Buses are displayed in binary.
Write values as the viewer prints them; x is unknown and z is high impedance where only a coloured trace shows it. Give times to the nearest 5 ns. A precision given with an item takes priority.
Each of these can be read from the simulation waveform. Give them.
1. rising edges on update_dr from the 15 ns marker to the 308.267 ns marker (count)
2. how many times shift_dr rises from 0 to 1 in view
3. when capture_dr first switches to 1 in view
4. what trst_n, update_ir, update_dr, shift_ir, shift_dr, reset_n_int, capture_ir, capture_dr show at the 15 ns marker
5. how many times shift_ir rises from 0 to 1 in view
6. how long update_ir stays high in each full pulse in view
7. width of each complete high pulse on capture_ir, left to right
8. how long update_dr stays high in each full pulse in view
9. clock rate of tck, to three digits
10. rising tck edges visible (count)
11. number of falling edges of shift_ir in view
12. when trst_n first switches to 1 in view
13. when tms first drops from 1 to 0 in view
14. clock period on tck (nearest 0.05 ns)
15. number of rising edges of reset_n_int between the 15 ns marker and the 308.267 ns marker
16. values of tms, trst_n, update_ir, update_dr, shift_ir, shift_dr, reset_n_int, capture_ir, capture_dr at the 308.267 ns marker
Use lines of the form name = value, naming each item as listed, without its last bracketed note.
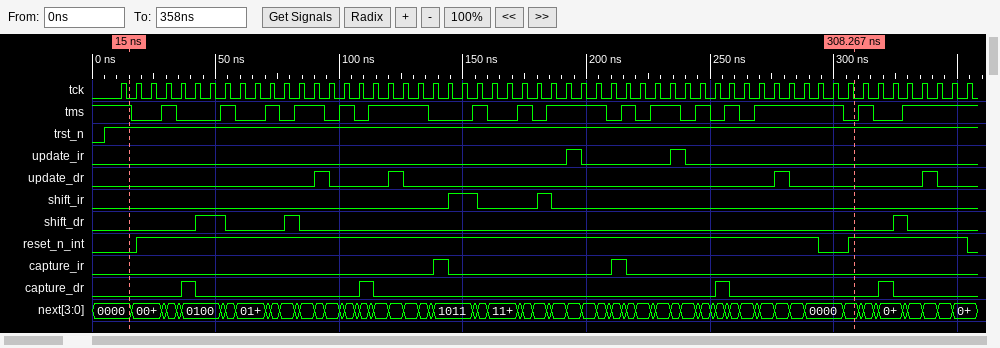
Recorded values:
rising edges on update_dr from the 15 ns marker to the 308.267 ns marker = 3
how many times shift_dr rises from 0 to 1 in view = 3
when capture_dr first switches to 1 in view = 35 ns
what trst_n, update_ir, update_dr, shift_ir, shift_dr, reset_n_int, capture_ir, capture_dr show at the 15 ns marker = trst_n=1, update_ir=0, update_dr=0, shift_ir=0, shift_dr=0, reset_n_int=0, capture_ir=0, capture_dr=0
how many times shift_ir rises from 0 to 1 in view = 2
how long update_ir stays high in each full pulse in view = 5 ns, 5 ns
width of each complete high pulse on capture_ir, left to right = 5 ns, 5 ns
how long update_dr stays high in each full pulse in view = 5 ns, 5 ns, 5 ns, 5 ns
clock rate of tck, to three digits = 167 MHz
rising tck edges visible = 58
number of falling edges of shift_ir in view = 2
when trst_n first switches to 1 in view = 5 ns
when tms first drops from 1 to 0 in view = 15 ns
clock period on tck = 6 ns
number of rising edges of reset_n_int between the 15 ns marker and the 308.267 ns marker = 2
values of tms, trst_n, update_ir, update_dr, shift_ir, shift_dr, reset_n_int, capture_ir, capture_dr at the 308.267 ns marker = tms=0, trst_n=1, update_ir=0, update_dr=0, shift_ir=0, shift_dr=0, reset_n_int=1, capture_ir=0, capture_dr=0
